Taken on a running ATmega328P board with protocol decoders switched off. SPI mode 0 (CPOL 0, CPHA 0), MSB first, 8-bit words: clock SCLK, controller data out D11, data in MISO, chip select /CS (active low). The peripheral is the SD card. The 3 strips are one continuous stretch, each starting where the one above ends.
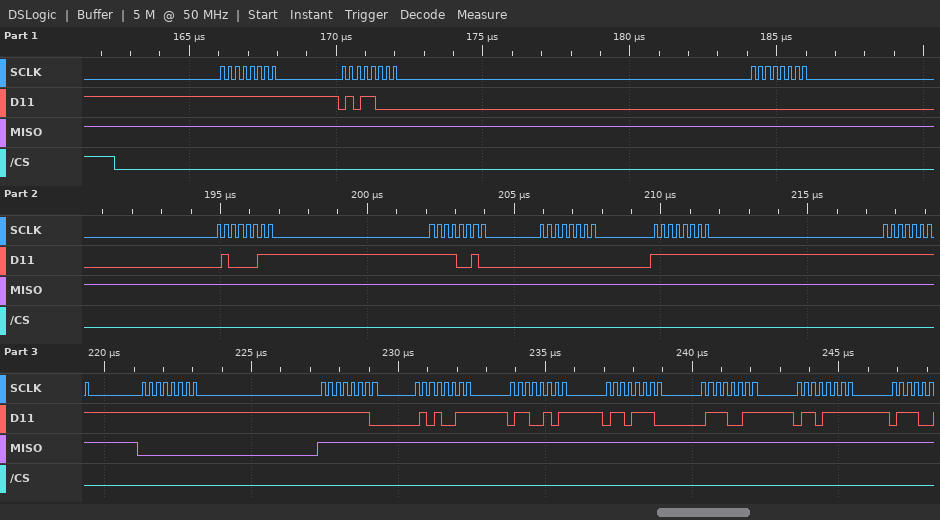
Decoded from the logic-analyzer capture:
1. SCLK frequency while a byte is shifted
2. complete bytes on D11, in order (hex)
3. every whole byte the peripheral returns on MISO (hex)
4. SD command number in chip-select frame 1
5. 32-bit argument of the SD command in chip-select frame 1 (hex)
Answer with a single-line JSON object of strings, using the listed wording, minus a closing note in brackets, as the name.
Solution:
{"SCLK frequency while a byte is shifted": "4 MHz", "complete bytes on D11, in order": "FF 58 00 43 F2 00 FF FF FF FE 53 65 6E 73 6F", "every whole byte the peripheral returns on MISO": "FF FF FF FF FF FF FF FF 00 FF FF FF FF FF FF", "SD command number in chip-select frame 1": "CMD24", "32-bit argument of the SD command in chip-select frame 1": "0x0043F200"}
